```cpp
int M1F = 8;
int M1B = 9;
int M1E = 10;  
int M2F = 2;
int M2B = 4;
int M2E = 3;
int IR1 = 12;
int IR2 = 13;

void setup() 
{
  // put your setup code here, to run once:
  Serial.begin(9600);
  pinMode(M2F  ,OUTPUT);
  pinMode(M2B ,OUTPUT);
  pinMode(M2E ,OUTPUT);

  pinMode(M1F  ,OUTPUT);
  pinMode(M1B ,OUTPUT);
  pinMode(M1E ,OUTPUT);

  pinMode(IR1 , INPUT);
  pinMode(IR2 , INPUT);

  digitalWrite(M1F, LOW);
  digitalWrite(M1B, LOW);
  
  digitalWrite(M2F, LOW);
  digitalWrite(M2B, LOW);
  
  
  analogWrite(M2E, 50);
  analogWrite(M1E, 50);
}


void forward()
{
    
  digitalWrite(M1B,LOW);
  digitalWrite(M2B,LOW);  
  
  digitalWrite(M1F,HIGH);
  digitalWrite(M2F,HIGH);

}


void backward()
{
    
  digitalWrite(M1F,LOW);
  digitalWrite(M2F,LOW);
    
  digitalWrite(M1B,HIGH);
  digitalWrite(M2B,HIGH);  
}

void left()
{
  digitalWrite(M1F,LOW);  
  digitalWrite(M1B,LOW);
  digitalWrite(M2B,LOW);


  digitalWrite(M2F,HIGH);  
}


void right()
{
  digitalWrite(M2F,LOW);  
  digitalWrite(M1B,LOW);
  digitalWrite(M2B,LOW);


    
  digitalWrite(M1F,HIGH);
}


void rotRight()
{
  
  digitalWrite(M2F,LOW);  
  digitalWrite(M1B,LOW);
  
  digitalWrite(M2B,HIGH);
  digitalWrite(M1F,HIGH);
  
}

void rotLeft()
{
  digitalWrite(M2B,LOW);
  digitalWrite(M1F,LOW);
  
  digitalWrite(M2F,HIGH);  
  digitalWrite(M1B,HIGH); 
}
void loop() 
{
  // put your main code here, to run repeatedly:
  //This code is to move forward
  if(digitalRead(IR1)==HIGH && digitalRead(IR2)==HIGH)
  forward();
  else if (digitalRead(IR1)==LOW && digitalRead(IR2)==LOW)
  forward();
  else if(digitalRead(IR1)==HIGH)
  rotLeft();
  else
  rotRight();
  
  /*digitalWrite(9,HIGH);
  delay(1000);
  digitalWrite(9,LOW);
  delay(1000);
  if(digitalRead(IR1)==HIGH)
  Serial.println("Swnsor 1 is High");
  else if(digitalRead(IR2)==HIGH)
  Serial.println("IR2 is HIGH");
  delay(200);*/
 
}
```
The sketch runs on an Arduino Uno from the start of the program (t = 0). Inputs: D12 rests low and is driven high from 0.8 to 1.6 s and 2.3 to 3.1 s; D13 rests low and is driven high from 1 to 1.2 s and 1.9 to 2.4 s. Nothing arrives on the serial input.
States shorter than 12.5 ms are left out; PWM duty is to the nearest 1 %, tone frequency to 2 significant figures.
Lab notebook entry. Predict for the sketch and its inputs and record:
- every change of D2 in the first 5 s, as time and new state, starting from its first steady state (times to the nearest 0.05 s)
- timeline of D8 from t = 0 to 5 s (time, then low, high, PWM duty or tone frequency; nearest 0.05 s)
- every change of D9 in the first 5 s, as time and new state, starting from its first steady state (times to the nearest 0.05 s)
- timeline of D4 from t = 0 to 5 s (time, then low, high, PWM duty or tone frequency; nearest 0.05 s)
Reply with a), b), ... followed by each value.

a) 0 s high; 1.9 s low; 2.3 s high
b) 0 s high; 0.8 s low; 1 s high; 1.2 s low; 1.6 s high; 2.4 s low; 3.1 s high
c) 0 s low; 0.8 s high; 1 s low; 1.2 s high; 1.6 s low; 2.4 s high; 3.1 s low
d) 0 s low; 1.9 s high; 2.3 s low
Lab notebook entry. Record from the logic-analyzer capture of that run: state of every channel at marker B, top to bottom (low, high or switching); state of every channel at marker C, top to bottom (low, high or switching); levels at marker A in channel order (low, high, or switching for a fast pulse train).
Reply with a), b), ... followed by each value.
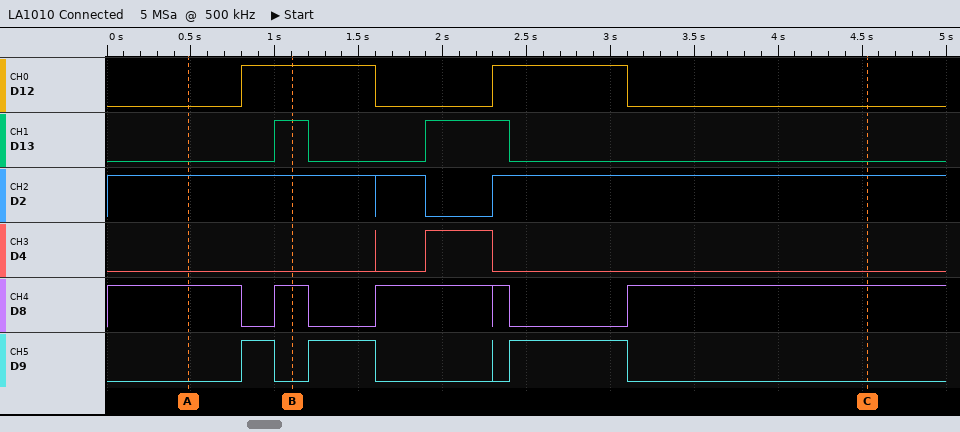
a) D12 high, D13 high, D2 high, D4 low, D8 high, D9 low
b) D12 low, D13 low, D2 high, D4 low, D8 high, D9 low
c) D12 low, D13 low, D2 high, D4 low, D8 high, D9 low
